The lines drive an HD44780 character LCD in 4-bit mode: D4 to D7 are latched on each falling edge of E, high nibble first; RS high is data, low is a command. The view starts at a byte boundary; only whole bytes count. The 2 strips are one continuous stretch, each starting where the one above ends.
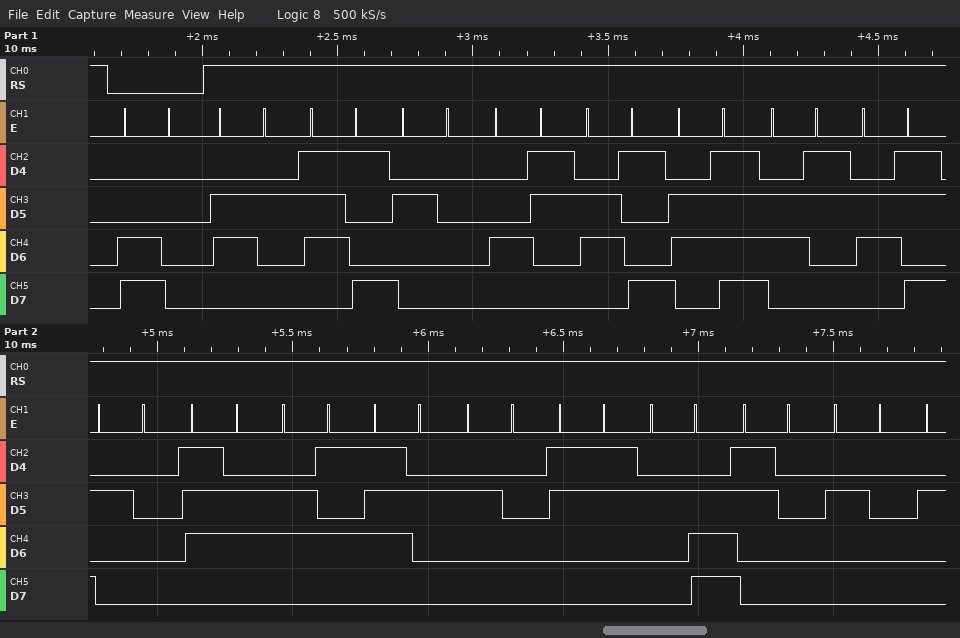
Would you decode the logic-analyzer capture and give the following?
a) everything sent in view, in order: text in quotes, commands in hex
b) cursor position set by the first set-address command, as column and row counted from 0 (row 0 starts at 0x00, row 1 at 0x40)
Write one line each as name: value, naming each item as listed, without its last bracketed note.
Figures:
everything sent in view, in order: text in quotes, commands in hex: 0xC0 "by Ciock ver 3.0 "
cursor position set by the first set-address command, as column and row counted from 0: column 0, row 1
